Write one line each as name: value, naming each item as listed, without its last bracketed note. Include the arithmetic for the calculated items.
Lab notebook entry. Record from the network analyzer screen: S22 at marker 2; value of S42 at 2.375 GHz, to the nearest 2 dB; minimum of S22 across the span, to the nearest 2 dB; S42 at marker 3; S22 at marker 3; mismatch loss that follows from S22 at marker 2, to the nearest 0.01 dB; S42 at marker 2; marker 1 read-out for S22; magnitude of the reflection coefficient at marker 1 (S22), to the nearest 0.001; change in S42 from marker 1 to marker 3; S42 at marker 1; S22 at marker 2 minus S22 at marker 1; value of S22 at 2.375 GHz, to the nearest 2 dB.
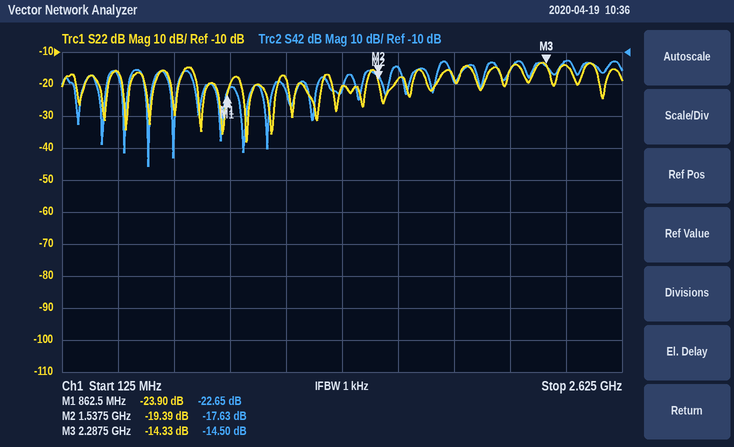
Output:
S22 at marker 2: -19.39 dB
value of S42 at 2.375 GHz, to the nearest 2 dB: -12 dB
minimum of S22 across the span, to the nearest 2 dB: -38 dB
S42 at marker 3: -14.50 dB
S22 at marker 3: -14.33 dB
mismatch loss that follows from S22 at marker 2, to the nearest 0.01 dB: −10 log10(1 − 10^(-19.39/10)) ≈ 0.05 dB
S42 at marker 2: -17.63 dB
marker 1 read-out for S22: -23.90 dB
magnitude of the reflection coefficient at marker 1 (S22), to the nearest 0.001: 10^(-23.9/20) ≈ 0.064
change in S42 from marker 1 to marker 3: -14.5 − (-22.65) = 8.15 dB
S42 at marker 1: -22.65 dB
S22 at marker 2 minus S22 at marker 1: -19.39 − (-23.9) = 4.51 dB
value of S22 at 2.375 GHz, to the nearest 2 dB: -14 dB
